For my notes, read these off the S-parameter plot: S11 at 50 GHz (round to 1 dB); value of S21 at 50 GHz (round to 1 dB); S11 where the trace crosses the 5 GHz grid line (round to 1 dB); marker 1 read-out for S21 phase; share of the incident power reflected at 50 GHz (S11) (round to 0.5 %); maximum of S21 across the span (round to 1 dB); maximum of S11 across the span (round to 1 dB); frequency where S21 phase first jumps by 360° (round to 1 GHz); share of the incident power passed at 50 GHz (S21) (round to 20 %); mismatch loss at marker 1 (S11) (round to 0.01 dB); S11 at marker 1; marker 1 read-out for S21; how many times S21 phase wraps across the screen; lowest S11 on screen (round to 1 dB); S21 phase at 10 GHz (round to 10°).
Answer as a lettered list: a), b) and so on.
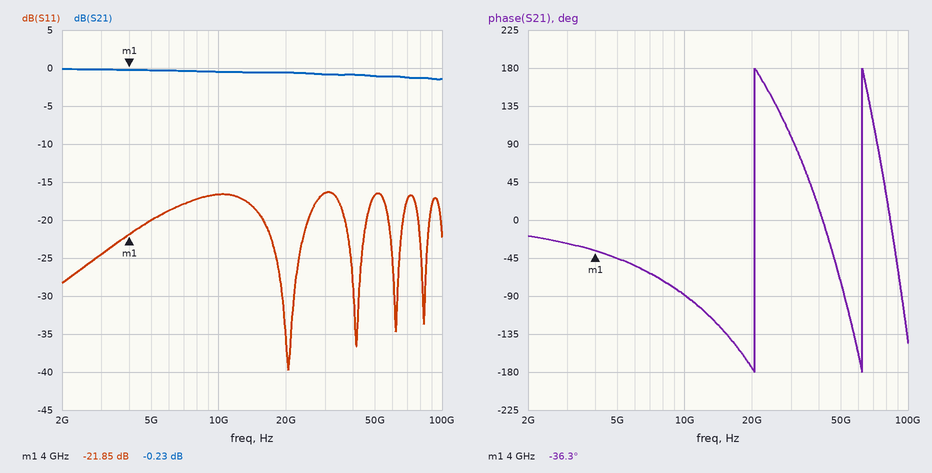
a) -17 dB
b) -1 dB
c) -20 dB
d) -36.3°
e) 2.0 %
f) 0 dB
g) -16 dB
h) 21 GHz
i) 80 %
j) 0.03 dB
k) -21.85 dB
l) -0.23 dB
m) 2
n) -40 dB
o) -90°
